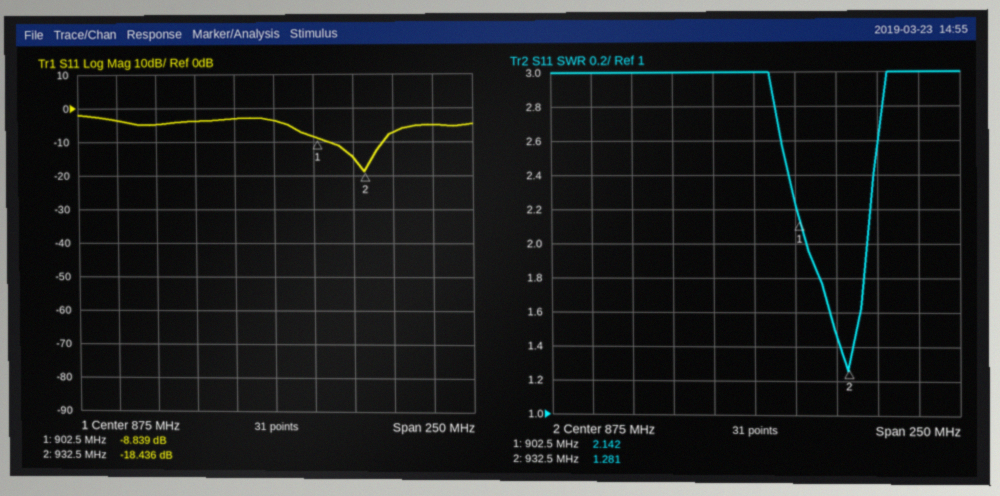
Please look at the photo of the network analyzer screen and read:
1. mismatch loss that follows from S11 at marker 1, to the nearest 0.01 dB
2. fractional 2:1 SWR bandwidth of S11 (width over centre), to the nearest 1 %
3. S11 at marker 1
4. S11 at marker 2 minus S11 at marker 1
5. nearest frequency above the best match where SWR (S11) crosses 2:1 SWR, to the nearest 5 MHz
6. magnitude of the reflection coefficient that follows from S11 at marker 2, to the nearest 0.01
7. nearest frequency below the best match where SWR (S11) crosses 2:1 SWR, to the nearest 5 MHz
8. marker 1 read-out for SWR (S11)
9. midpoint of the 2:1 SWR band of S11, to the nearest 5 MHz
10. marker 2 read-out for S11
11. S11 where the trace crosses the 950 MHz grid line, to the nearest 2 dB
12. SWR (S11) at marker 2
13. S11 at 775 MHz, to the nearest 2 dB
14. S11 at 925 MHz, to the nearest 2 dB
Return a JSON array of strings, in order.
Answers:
["0.61 dB", "4 %", "-8.839 dB", "-9.597 dB", "945 MHz", "0.12", "905 MHz", "2.142", "925 MHz", "-18.436 dB", "-8 dB", "1.281", "-4 dB", "-14 dB"]
